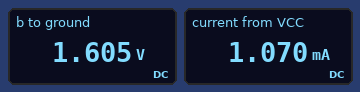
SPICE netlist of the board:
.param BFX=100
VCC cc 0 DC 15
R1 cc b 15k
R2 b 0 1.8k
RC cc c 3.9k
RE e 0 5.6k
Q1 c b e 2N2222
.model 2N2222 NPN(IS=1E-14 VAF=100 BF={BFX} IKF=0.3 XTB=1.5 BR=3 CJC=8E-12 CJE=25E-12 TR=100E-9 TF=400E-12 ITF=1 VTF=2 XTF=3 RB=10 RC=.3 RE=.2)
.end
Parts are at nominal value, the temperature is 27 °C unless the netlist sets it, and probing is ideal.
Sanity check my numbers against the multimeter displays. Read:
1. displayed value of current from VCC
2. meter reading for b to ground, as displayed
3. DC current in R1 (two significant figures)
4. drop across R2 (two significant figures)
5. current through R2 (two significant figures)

1.070 mA
1.605 V
890 µA
1.6 V
890 µA
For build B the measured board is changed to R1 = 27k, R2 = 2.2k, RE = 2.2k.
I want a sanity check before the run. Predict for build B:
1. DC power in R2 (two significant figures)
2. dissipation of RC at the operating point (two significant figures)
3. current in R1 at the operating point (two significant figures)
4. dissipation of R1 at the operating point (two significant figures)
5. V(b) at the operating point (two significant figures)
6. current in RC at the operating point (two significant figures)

580 µW
210 µW
510 µA
7.1 mW
1.1 V
230 µA
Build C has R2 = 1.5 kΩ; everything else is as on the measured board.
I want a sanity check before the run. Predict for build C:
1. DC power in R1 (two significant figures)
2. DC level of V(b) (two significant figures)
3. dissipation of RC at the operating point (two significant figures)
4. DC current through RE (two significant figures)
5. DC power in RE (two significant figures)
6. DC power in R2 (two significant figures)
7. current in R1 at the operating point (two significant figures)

12 mW
1.4 V
71 µW
140 µA
100 µW
1.2 mW
910 µA
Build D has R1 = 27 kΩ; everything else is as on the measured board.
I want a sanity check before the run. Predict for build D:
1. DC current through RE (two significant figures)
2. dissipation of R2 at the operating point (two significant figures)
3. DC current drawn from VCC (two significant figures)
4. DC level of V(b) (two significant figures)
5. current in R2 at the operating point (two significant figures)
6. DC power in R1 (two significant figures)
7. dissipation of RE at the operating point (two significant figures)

64 µA
490 µW
580 µA
940 mV
520 µA
7.3 mW
23 µW
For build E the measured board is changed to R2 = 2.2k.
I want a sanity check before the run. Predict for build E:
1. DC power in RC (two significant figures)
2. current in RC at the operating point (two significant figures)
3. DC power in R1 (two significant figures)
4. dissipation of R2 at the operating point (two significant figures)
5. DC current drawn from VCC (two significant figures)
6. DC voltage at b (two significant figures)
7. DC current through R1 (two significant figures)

210 µW
230 µA
11 mW
1.7 mW
1.1 mA
1.9 V
870 µA
